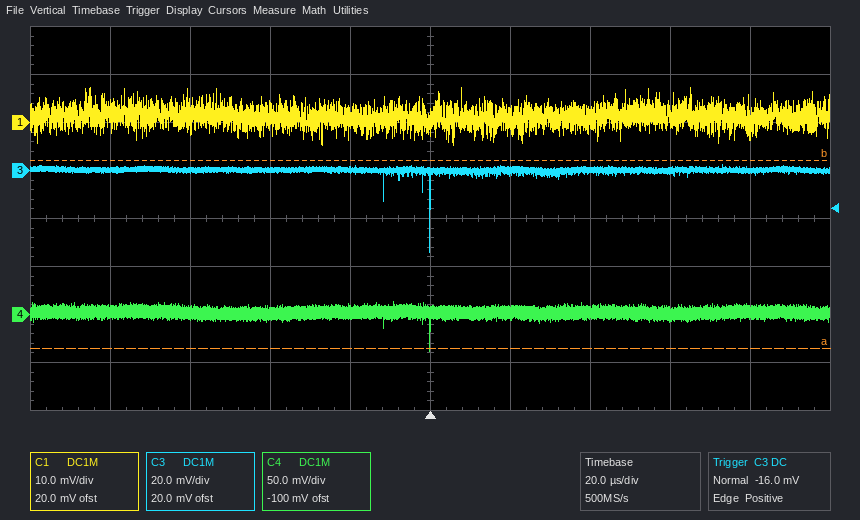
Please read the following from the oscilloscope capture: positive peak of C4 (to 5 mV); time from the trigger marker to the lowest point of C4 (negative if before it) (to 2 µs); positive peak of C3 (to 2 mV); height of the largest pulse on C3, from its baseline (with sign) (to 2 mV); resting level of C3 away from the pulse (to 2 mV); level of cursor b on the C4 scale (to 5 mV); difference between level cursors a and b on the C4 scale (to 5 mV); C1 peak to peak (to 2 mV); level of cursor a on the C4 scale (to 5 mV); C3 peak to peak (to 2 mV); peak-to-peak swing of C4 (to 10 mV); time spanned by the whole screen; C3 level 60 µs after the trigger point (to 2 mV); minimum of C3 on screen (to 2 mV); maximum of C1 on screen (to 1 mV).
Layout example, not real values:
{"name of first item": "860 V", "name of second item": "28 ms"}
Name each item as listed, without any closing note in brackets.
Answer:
{"positive peak of C4": "15 mV", "time from the trigger marker to the lowest point of C4 (negative if before it)": "0 µs", "positive peak of C3": "2 mV", "height of the largest pulse on C3, from its baseline (with sign)": "-34 mV", "resting level of C3 away from the pulse": "0 mV", "level of cursor b on the C4 scale": "160 mV", "difference between level cursors a and b on the C4 scale": "195 mV", "C1 peak to peak": "12 mV", "level of cursor a on the C4 scale": "-35 mV", "C3 peak to peak": "36 mV", "peak-to-peak swing of C4": "50 mV", "time spanned by the whole screen": "200 µs", "C3 level 60 µs after the trigger point": "0 mV", "minimum of C3 on screen": "-34 mV", "maximum of C1 on screen": "7 mV"}
